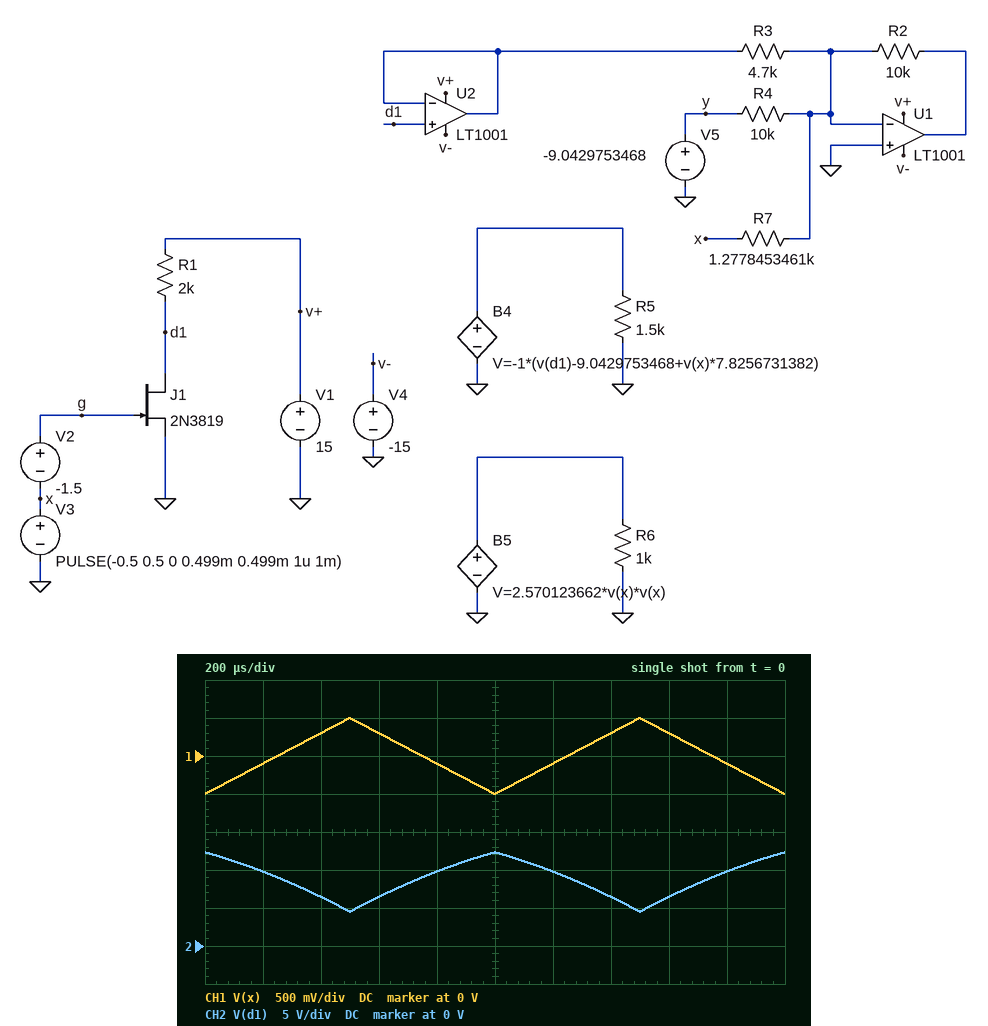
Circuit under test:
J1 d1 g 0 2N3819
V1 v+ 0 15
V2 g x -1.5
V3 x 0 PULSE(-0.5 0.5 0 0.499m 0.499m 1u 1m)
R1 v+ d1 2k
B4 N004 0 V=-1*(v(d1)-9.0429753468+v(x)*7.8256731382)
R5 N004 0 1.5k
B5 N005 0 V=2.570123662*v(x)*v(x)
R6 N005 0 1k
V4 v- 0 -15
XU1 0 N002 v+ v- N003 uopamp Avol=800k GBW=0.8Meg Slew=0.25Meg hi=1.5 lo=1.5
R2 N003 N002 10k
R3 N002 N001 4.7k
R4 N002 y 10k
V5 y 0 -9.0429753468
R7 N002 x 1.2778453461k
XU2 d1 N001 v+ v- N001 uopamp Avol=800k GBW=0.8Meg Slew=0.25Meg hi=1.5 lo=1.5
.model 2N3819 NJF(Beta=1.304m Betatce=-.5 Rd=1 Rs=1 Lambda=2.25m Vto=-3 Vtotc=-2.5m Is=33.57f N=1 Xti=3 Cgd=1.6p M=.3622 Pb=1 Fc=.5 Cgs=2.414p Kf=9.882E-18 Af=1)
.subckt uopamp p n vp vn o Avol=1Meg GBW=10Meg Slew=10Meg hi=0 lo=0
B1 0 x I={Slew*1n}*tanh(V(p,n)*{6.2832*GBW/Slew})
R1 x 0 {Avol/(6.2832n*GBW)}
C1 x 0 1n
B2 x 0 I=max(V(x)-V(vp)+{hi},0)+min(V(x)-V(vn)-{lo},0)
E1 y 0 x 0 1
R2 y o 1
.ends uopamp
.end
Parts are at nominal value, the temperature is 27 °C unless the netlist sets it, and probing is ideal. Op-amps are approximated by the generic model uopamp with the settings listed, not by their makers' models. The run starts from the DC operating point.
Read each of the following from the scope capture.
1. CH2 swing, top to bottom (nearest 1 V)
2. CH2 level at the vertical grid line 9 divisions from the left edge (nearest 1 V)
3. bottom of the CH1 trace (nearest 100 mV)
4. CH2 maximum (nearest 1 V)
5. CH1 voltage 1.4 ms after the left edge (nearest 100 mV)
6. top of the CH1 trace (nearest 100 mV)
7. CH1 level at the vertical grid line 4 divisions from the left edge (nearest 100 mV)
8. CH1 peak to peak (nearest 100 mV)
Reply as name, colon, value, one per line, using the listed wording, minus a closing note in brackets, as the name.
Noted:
CH2 swing, top to bottom: 8 V
CH2 level at the vertical grid line 9 divisions from the left edge: 10 V
bottom of the CH1 trace: -500 mV
CH2 maximum: 12 V
CH1 voltage 1.4 ms after the left edge: 300 mV
top of the CH1 trace: 500 mV
CH1 level at the vertical grid line 4 divisions from the left edge: -100 mV
CH1 peak to peak: 1.0 V
